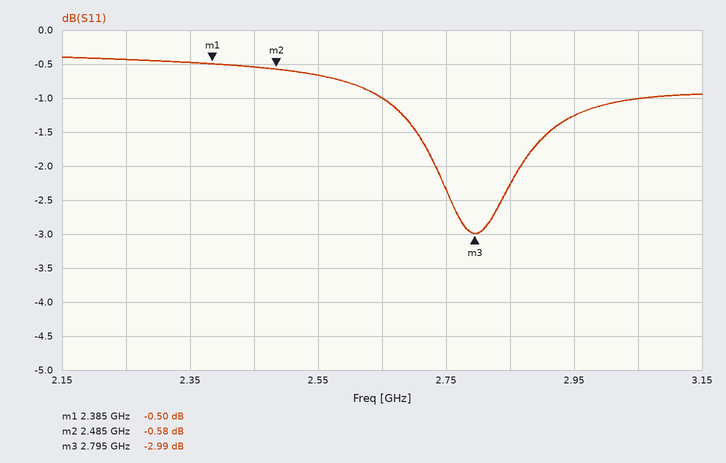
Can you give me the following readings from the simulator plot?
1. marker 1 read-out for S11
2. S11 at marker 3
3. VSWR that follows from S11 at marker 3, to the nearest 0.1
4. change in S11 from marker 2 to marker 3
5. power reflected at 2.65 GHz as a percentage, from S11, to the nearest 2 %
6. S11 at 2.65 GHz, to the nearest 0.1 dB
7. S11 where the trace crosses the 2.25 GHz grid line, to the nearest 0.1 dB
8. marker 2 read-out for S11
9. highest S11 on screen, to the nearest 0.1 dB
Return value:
-0.50 dB
-2.99 dB
5.9
-2.41 dB
80 %
-1.0 dB
-0.4 dB
-0.58 dB
-0.4 dB
